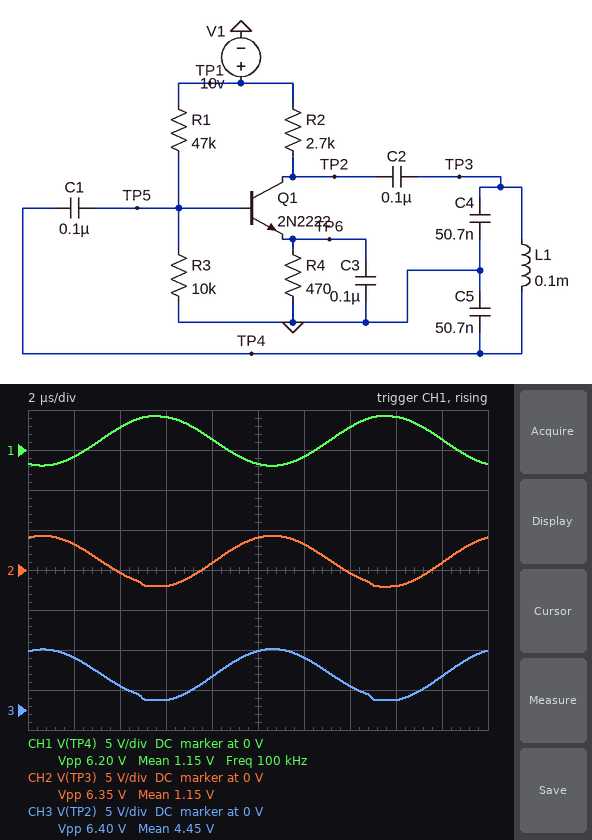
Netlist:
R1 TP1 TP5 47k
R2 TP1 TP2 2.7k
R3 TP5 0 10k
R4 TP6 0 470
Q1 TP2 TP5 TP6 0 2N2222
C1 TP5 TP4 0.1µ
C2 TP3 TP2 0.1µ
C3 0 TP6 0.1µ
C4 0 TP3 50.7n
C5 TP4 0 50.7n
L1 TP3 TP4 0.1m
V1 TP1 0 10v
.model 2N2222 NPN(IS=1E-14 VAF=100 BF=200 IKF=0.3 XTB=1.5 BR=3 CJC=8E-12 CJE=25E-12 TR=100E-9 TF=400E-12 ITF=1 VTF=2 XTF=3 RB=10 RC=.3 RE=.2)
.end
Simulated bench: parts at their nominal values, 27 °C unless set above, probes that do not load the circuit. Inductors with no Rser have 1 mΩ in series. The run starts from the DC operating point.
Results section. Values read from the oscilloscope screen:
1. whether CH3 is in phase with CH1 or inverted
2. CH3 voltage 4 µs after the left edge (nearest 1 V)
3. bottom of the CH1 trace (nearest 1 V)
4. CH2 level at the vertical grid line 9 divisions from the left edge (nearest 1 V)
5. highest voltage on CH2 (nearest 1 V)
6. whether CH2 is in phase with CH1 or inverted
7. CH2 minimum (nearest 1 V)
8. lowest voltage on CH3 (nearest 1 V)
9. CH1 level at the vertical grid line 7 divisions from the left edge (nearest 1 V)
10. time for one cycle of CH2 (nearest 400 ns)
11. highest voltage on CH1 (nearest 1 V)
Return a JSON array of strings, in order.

["inverted", "3 V", "-2 V", "1 V", "4 V", "inverted", "-2 V", "1 V", "3 V", "10.0 µs", "4 V"]
